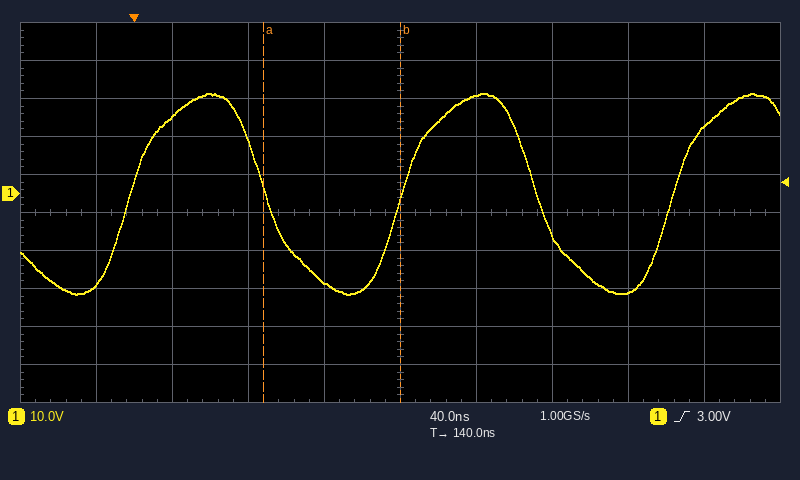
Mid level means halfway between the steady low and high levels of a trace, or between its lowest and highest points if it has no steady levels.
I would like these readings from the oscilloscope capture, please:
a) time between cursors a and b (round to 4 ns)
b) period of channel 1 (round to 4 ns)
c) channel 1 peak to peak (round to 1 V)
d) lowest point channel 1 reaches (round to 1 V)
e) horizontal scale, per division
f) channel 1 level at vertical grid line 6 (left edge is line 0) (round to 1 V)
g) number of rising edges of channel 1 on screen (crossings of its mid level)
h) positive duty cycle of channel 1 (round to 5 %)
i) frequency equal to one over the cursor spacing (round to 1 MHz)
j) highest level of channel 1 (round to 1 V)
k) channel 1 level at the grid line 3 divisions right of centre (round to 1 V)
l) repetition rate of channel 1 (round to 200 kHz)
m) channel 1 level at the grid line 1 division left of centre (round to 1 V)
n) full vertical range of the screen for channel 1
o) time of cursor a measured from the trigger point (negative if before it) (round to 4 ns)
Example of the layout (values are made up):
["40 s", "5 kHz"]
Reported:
["72 ns", "144 ns", "53 V", "-27 V", "40 ns", "26 V", "3", "50 %", "14 MHz", "26 V", "-26 V", "7.0 MHz", "-23 V", "100 V", "+68 ns"]
